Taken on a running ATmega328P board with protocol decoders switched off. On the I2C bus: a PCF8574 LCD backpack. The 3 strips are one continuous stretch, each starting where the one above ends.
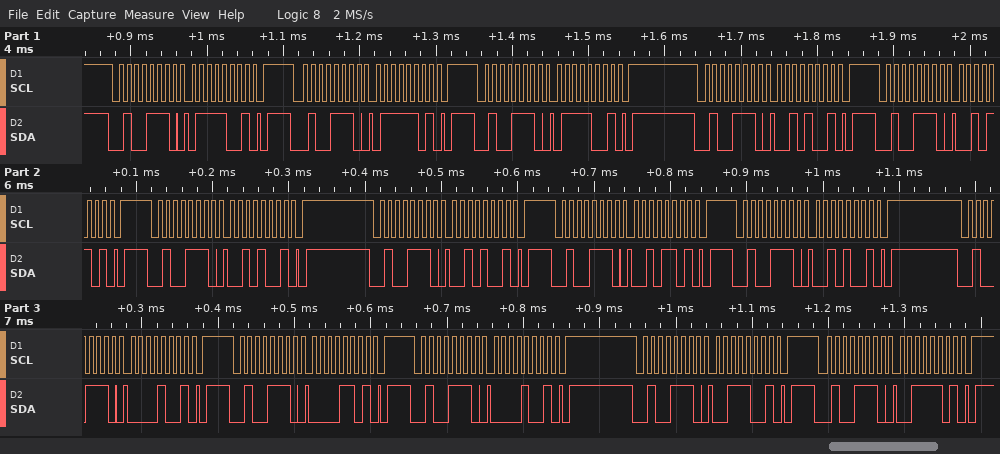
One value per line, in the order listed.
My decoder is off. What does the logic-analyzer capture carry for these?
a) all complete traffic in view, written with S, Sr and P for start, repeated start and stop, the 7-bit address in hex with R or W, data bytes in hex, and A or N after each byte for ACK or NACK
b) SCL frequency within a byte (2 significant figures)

S 27W A 79 A P S 27W A 7D A P S 27W A 79 A P S 27W A 29 A P S 27W A 2D A P S 27W A 29 A P S 27W A 29 A P S 27W A 2D A P S 27W A 29 A P S 27W A 09 A P S 27W A 0D A P S 27W A 09 A P S 27W A 39 A P S 27W A 3D A P
100 kHz
